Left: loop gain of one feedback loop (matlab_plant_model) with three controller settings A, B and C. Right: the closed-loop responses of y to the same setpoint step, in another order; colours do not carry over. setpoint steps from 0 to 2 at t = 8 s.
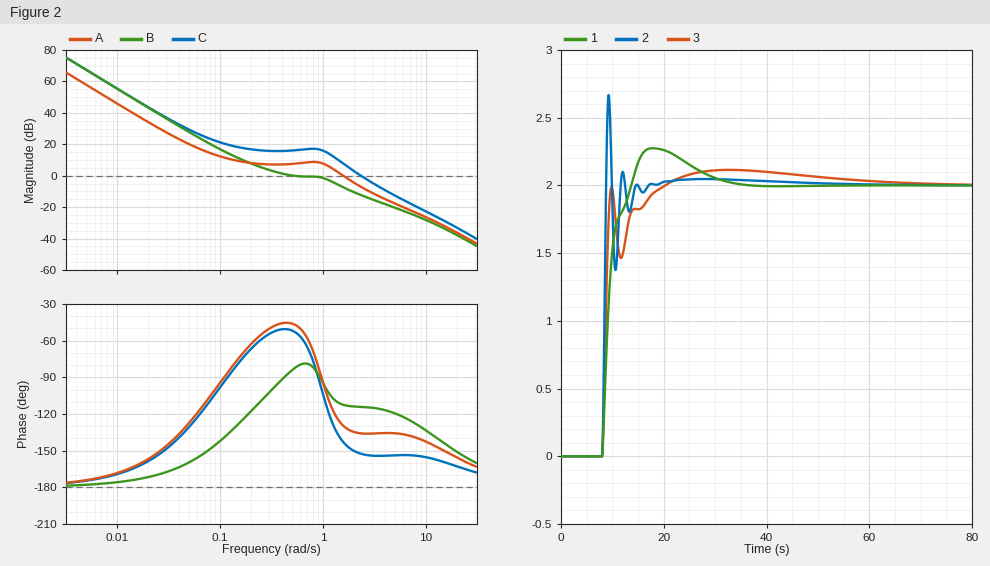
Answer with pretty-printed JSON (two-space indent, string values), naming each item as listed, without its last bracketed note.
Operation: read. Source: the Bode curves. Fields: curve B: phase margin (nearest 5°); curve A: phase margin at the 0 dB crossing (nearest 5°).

{
  "curve B: phase margin": "95°",
  "curve A: phase margin at the 0 dB crossing": "50°"
}
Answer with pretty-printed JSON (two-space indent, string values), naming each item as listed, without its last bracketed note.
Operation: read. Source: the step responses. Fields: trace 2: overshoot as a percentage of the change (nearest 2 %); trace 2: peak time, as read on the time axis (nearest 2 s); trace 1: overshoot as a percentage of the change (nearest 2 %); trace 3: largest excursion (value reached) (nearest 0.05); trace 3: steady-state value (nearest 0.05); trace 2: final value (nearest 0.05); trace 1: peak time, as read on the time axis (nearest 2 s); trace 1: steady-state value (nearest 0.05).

{
  "trace 2: overshoot as a percentage of the change": "34 %",
  "trace 2: peak time, as read on the time axis": "10 s",
  "trace 1: overshoot as a percentage of the change": "14 %",
  "trace 3: largest excursion (value reached)": "2.10",
  "trace 3: steady-state value": "2.00",
  "trace 2: final value": "2.00",
  "trace 1: peak time, as read on the time axis": "18 s",
  "trace 1: steady-state value": "2.00"
}
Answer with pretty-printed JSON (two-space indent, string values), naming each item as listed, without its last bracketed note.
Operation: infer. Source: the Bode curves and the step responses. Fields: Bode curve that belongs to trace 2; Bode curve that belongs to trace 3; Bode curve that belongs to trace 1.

{
  "Bode curve that belongs to trace 2": "C",
  "Bode curve that belongs to trace 3": "A",
  "Bode curve that belongs to trace 1": "B"
}
